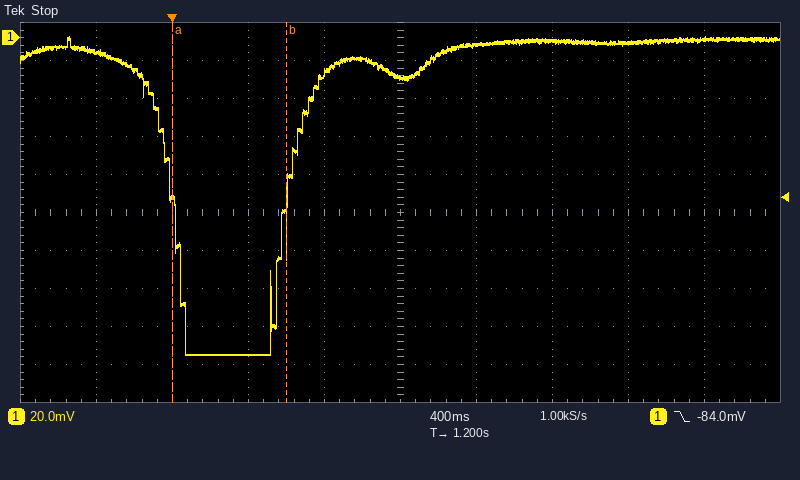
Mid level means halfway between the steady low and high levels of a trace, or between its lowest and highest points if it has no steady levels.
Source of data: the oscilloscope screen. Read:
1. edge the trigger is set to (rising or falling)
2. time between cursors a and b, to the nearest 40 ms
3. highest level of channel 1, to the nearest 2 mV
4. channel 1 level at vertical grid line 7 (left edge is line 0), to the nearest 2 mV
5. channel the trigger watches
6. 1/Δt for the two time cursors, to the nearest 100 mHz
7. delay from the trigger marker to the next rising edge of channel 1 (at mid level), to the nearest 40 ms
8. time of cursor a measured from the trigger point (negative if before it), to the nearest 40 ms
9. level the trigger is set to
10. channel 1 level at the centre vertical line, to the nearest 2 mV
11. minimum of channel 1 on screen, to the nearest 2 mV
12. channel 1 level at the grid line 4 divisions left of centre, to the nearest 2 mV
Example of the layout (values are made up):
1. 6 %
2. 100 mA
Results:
1. falling
2. 600 ms
3. 0 mV
4. -2 mV
5. channel 1
6. 1.7 Hz
7. 600 ms
8. 0 ms
9. -84.0 mV
10. -20 mV
11. -166 mV
12. -8 mV
